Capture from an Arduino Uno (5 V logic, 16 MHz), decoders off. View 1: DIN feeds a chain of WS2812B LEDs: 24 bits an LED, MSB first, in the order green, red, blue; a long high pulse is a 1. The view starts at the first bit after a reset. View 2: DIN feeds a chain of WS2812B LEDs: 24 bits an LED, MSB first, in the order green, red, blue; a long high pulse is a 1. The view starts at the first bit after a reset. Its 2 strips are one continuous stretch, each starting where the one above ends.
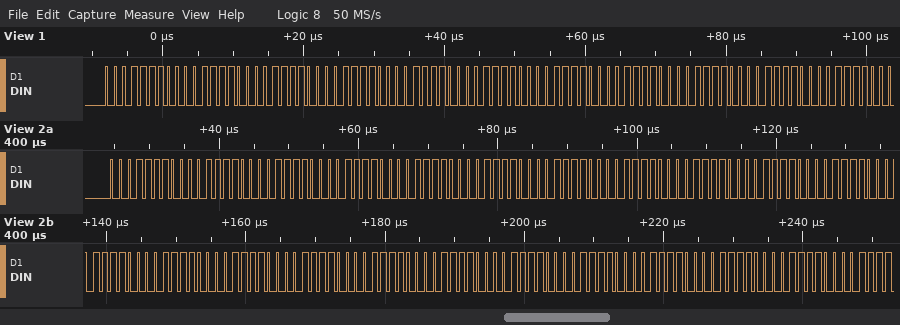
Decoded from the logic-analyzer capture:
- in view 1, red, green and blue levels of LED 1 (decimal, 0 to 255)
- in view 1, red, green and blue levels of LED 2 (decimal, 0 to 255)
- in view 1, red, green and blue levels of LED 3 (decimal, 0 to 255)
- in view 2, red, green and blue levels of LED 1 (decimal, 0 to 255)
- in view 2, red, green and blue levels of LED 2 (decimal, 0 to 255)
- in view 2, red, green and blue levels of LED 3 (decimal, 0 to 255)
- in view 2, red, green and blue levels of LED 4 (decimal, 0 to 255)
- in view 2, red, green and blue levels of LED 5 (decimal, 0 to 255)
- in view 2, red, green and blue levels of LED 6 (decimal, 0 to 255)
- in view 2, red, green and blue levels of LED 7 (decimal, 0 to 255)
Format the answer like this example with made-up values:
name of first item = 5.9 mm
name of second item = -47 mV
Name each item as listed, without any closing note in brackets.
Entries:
in view 1, red, green and blue levels of LED 1 = 30, 30, 30
in view 1, red, green and blue levels of LED 2 = 30, 30, 30
in view 1, red, green and blue levels of LED 3 = 30, 30, 30
in view 2, red, green and blue levels of LED 1 = 30, 30, 30
in view 2, red, green and blue levels of LED 2 = 30, 30, 30
in view 2, red, green and blue levels of LED 3 = 30, 30, 30
in view 2, red, green and blue levels of LED 4 = 30, 30, 30
in view 2, red, green and blue levels of LED 5 = 30, 30, 30
in view 2, red, green and blue levels of LED 6 = 30, 30, 30
in view 2, red, green and blue levels of LED 7 = 30, 30, 30
